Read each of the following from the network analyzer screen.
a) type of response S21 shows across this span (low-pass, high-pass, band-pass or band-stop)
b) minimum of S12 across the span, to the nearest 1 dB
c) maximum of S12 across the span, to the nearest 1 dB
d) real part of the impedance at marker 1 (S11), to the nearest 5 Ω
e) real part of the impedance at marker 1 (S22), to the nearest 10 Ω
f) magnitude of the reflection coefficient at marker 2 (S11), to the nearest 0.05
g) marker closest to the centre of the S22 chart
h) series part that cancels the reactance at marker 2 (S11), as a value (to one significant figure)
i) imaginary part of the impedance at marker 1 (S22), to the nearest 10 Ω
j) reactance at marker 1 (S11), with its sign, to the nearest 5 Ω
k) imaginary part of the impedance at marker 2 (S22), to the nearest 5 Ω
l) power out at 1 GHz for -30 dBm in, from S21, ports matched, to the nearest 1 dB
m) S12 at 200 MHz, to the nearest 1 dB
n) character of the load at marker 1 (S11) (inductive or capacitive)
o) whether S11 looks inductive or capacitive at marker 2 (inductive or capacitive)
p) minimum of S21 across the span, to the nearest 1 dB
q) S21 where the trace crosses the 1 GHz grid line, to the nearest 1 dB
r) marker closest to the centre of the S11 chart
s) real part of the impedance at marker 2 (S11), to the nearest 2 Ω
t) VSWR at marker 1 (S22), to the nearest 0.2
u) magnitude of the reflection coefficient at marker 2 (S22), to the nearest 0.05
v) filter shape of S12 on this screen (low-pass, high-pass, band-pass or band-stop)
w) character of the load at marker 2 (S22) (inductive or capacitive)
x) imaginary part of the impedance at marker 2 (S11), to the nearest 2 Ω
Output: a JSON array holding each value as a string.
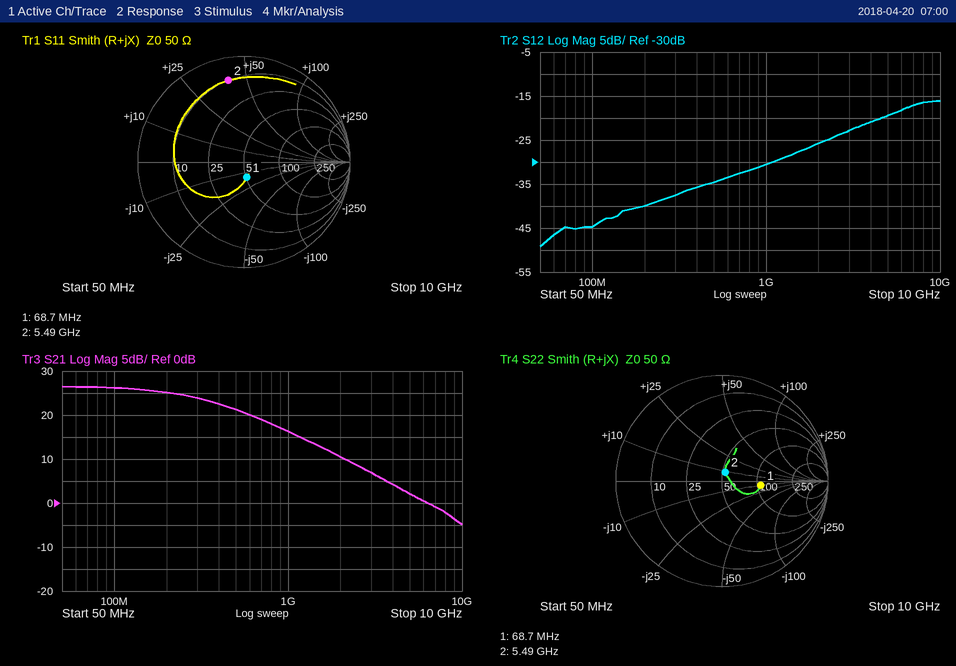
["low-pass", "-49 dB", "-16 dB", "50 Ω", "110 Ω", "0.80", "marker 2", "700 fF", "-10 Ω", "-15 Ω", "+10 Ω", "-14 dBm", "-40 dB", "capacitive", "inductive", "-5 dB", "16 dB", "marker 1", "10 Ω", "2.2", "0.10", "high-pass", "inductive", "+40 Ω"]
